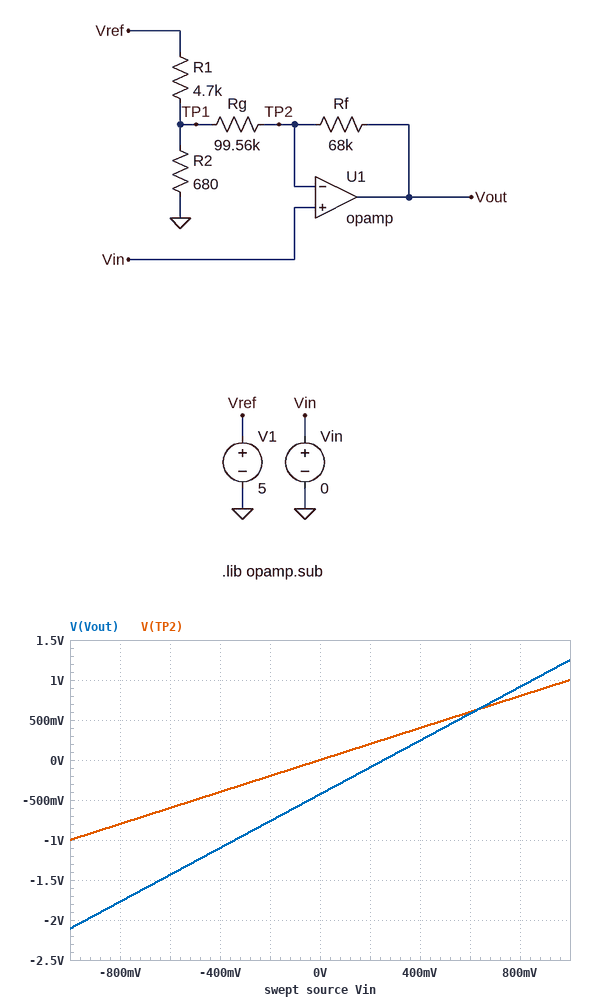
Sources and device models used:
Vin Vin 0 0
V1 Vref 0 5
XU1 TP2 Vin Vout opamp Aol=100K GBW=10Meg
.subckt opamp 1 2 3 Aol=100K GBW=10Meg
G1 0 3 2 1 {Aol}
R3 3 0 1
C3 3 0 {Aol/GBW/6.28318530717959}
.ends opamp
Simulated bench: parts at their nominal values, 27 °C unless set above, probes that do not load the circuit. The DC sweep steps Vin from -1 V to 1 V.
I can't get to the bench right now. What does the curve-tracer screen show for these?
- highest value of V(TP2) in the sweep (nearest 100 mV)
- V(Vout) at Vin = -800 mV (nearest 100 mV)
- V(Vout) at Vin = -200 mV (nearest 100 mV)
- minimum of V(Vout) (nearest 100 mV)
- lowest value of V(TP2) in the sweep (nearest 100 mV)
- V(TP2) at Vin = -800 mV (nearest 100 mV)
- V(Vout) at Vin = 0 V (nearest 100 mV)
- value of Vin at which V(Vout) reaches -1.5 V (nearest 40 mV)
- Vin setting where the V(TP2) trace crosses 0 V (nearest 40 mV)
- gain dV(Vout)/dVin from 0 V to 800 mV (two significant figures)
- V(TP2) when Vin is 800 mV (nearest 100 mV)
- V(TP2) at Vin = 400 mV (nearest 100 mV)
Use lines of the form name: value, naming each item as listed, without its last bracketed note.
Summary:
highest value of V(TP2) in the sweep: 1.0 V
V(Vout) at Vin = -800 mV: -1.8 V
V(Vout) at Vin = -200 mV: -800 mV
minimum of V(Vout): -2.1 V
lowest value of V(TP2) in the sweep: -1.0 V
V(TP2) at Vin = -800 mV: -800 mV
V(Vout) at Vin = 0 V: -400 mV
value of Vin at which V(Vout) reaches -1.5 V: -640 mV
Vin setting where the V(TP2) trace crosses 0 V: 0 V
gain dV(Vout)/dVin from 0 V to 800 mV: 1.7 V/V
V(TP2) when Vin is 800 mV: 800 mV
V(TP2) at Vin = 400 mV: 400 mV
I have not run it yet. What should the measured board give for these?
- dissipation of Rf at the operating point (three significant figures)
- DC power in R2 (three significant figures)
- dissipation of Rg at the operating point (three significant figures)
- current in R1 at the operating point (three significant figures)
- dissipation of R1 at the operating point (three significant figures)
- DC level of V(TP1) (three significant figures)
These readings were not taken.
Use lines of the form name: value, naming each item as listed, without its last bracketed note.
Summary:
dissipation of Rf at the operating point: 2.71 µW
DC power in R2: 580 µW
dissipation of Rg at the operating point: 3.96 µW
current in R1 at the operating point: 930 µA
dissipation of R1 at the operating point: 4.07 mW
DC level of V(TP1): 628 mV
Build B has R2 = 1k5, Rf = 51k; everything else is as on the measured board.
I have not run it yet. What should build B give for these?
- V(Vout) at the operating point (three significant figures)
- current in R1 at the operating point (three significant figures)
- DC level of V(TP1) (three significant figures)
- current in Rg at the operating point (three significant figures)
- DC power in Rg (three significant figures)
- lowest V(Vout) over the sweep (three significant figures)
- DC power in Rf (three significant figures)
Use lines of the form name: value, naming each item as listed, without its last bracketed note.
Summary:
V(Vout) at the operating point: -613 mV
current in R1 at the operating point: 809 µA
DC level of V(TP1): 1.20 V
current in Rg at the operating point: 12.0 µA
DC power in Rg: 14.4 µW
lowest V(Vout) over the sweep: -2.12 V
DC power in Rf: 7.36 µW
